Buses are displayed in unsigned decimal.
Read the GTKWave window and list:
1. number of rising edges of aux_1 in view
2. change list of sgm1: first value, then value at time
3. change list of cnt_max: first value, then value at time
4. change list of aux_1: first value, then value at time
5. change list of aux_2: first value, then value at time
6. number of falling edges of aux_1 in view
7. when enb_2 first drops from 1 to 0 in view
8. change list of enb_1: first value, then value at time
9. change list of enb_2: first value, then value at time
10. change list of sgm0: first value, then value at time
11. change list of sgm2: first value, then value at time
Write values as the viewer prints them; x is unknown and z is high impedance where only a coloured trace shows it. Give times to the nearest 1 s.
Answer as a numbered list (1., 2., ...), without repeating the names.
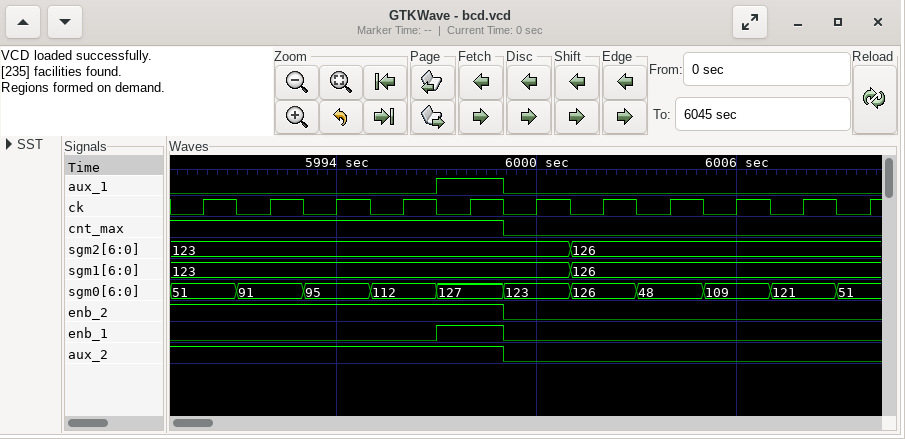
1. 1
2. 123, 126 at 6001 s
3. 1, 0 at 5999 s
4. 0, 1 at 5997 s, 0 at 5999 s
5. 1, 0 at 5999 s
6. 1
7. 5999 s
8. 0, 1 at 5997 s, 0 at 5999 s
9. 1, 0 at 5999 s
10. 51, 91 at 5991 s, 95 at 5993 s, 112 at 5995 s, 127 at 5997 s, 123 at 5999 s, 126 at 6001 s, 48 at 6003 s, 109 at 6005 s, 121 at 6007 s, 51 at 6009 s
11. 123, 126 at 6001 s
